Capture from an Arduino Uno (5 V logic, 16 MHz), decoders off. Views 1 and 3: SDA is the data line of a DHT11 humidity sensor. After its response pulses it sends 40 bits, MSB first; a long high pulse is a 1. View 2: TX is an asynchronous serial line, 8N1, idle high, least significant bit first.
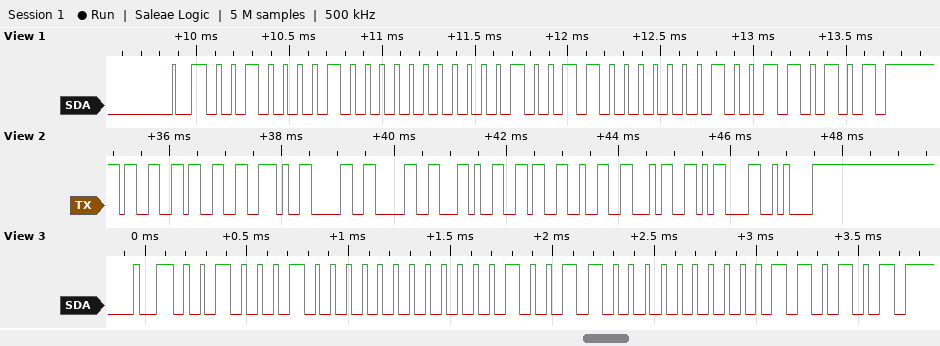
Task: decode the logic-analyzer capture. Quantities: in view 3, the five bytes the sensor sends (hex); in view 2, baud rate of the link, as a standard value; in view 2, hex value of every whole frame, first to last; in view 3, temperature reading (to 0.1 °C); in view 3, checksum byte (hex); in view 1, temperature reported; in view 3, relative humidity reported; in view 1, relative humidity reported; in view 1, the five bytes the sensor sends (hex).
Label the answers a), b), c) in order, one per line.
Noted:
a) 22 00 13 00 35
b) 9600 baud
c) 33 33 2E 30 30 2C 36 32 34 0D 0A
d) 19.0 °C
e) 0x35
f) 19.1 °C
g) 34 %
h) 33 %
i) 21 00 13 01 35
